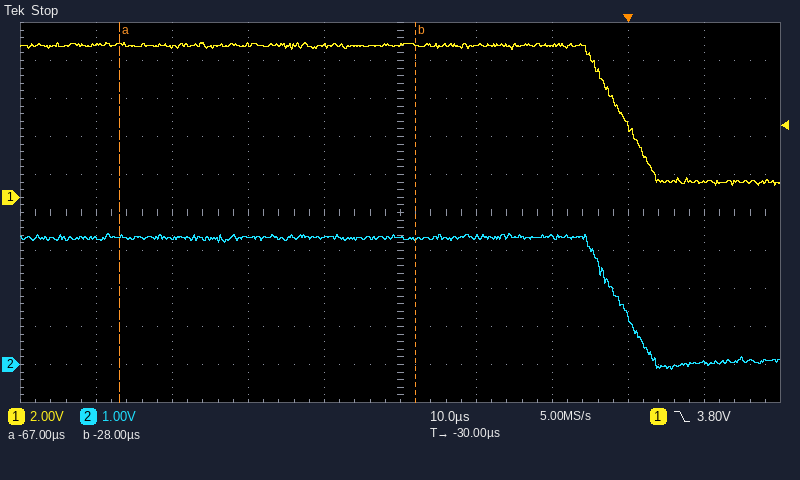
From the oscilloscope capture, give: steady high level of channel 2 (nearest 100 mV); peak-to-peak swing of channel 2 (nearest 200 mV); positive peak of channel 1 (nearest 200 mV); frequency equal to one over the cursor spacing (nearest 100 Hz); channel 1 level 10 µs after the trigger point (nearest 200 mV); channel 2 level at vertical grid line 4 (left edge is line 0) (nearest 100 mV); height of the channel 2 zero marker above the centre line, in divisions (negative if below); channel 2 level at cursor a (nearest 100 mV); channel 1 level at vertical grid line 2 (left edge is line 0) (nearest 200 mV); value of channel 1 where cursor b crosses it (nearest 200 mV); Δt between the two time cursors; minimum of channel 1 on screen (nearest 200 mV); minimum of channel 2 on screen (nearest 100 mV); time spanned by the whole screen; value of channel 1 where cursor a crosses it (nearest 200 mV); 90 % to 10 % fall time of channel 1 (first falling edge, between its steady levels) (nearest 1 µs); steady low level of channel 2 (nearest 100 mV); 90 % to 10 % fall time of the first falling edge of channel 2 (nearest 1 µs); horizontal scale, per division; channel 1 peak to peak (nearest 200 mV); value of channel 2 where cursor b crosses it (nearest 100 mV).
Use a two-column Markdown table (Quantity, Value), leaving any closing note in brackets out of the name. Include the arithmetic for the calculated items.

| Quantity | Value |
|---|---|
| steady high level of channel 2 | 3.3 V |
| peak-to-peak swing of channel 2 | 3.6 V |
| positive peak of channel 1 | 8.2 V |
| frequency equal to one over the cursor spacing | 1 / 39 µs ≈ 25.6 kHz |
| channel 1 level 10 µs after the trigger point | 800 mV |
| channel 2 level at vertical grid line 4 (left edge is line 0) | 3.3 V |
| height of the channel 2 zero marker above the centre line, in divisions | -4.0 div |
| channel 2 level at cursor a | 3.4 V |
| channel 1 level at vertical grid line 2 (left edge is line 0) | 8.0 V |
| value of channel 1 where cursor b crosses it | 8.0 V |
| Δt between the two time cursors | -28 µs − (-67 µs) = 39 µs |
| minimum of channel 1 on screen | 600 mV |
| minimum of channel 2 on screen | -100 mV |
| time spanned by the whole screen | 100 µs |
| value of channel 1 where cursor a crosses it | 8.0 V |
| 90 % to 10 % fall time of channel 1 (first falling edge, between its steady levels) | 8 µs |
| steady low level of channel 2 | 100 mV |
| 90 % to 10 % fall time of the first falling edge of channel 2 | 7 µs |
| horizontal scale, per division | 10 µs |
| channel 1 peak to peak | 8.2 V − (600 mV) = 7.6 V |
| value of channel 2 where cursor b crosses it | 3.3 V |
